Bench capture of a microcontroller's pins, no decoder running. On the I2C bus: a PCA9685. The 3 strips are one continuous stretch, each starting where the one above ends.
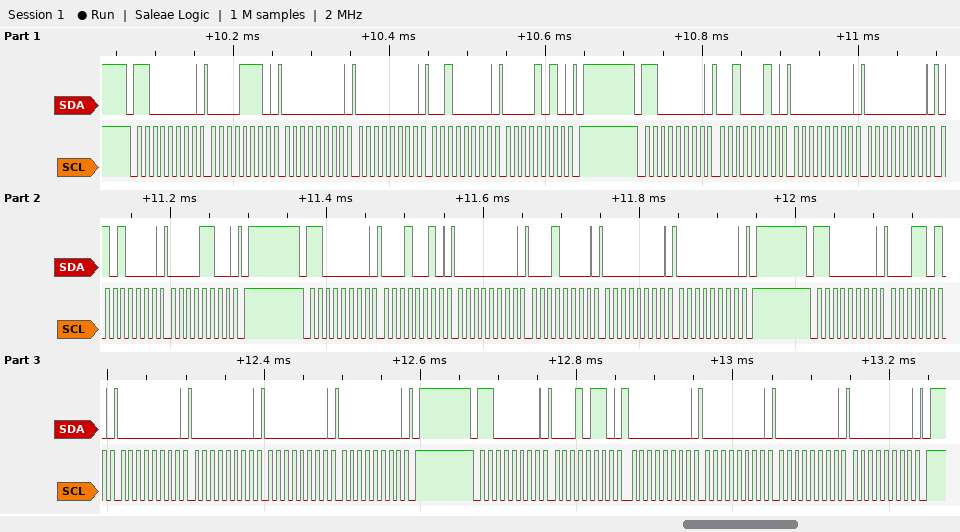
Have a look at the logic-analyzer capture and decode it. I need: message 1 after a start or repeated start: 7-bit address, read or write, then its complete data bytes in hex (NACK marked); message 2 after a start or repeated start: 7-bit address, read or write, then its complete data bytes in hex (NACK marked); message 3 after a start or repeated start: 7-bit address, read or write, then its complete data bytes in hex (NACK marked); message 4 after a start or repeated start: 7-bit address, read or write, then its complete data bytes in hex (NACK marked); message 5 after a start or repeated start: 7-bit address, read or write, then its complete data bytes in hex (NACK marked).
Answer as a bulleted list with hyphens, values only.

- 0x60 write: 0E 00 00 20 0A
- 0x60 write: 22 00 00 50 0C
- 0x60 write: 12 00 10 00 00
- 0x60 write: 1A 00 00 00 00
- 0x60 write: 16 00 00 00 00
